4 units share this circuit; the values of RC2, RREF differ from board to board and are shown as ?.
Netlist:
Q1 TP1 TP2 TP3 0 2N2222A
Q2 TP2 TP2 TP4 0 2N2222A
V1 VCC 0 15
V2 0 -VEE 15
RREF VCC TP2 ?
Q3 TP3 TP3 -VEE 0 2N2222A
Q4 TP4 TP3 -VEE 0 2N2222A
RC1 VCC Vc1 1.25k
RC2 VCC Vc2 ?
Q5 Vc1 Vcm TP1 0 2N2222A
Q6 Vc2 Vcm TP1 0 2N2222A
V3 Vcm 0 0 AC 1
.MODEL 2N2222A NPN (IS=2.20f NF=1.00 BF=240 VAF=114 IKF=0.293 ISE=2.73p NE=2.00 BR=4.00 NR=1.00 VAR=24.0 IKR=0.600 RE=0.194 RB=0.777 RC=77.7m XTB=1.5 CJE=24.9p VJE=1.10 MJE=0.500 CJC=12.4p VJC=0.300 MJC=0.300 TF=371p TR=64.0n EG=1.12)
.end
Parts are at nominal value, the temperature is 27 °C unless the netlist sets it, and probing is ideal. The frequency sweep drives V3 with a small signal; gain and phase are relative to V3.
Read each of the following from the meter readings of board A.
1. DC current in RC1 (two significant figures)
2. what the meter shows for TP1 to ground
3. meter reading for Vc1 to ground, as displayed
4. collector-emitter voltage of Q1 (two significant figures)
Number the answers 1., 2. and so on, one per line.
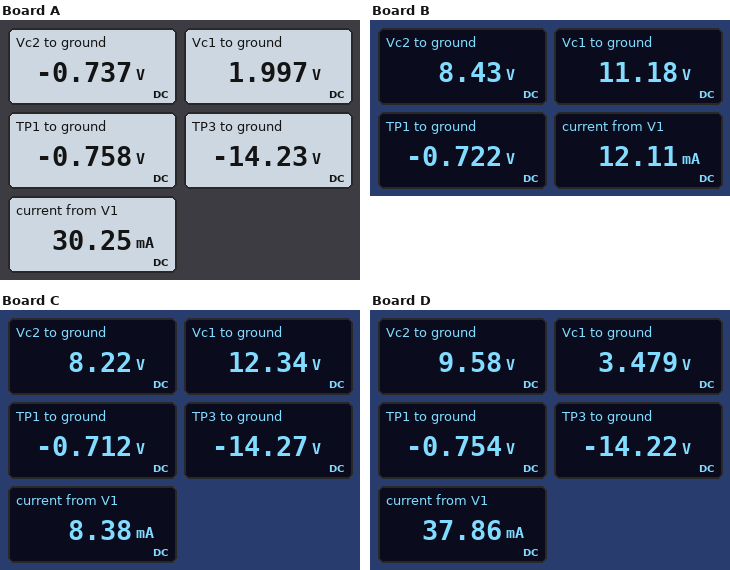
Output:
1. 10 mA
2. -0.758 V
3. 1.997 V
4. 13 V
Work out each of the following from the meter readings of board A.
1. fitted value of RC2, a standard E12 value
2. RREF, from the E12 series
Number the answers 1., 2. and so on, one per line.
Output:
1. 3.9 kΩ
2. 1.8 kΩ
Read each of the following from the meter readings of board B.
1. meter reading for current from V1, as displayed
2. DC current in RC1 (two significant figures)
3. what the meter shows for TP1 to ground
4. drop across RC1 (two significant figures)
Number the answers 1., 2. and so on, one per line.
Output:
1. 12.11 mA
2. 3.1 mA
3. -0.722 V
4. 3.8 V
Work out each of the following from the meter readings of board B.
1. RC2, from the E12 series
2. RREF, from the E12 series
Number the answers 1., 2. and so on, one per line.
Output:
1. 2.2 kΩ
2. 4.7 kΩ
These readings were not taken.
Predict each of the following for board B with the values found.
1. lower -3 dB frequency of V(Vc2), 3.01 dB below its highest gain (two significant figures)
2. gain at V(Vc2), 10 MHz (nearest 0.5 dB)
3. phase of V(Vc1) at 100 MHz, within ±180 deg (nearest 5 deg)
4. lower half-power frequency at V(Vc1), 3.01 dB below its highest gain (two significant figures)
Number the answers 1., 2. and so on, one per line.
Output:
1. 140 MHz
2. -23.0 dB
3. 85 deg
4. 140 MHz
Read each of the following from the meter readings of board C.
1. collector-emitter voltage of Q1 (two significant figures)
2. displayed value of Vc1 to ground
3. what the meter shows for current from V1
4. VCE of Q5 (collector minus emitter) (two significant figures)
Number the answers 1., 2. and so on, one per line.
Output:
1. 14 V
2. 12.34 V
3. 8.38 mA
4. 13 V
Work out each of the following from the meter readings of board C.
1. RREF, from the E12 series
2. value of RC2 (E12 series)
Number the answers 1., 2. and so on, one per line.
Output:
1. 6.8 kΩ
2. 3.3 kΩ
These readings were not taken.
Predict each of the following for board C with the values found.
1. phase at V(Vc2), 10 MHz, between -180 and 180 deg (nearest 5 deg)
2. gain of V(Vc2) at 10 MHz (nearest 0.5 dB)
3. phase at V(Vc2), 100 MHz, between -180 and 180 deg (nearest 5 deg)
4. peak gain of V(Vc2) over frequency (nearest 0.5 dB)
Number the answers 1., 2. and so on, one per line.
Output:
1. 65 deg
2. -20.0 dB
3. 60 deg
4. 0.5 dB
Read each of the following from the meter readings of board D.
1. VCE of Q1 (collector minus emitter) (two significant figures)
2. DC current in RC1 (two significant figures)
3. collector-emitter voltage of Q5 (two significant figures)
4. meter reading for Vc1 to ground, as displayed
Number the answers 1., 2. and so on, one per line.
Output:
1. 13 V
2. 9.2 mA
3. 4.2 V
4. 3.479 V
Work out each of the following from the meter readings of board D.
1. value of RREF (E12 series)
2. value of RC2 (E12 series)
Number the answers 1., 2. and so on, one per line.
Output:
1. 1.5 kΩ
2. 560 Ω
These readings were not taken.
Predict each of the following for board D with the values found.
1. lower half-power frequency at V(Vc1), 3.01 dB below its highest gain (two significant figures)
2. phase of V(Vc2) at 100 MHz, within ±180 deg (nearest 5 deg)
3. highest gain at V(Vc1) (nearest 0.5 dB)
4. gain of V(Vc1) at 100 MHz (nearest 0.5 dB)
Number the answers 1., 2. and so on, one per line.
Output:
1. 200 MHz
2. 105 deg
3. 0 dB
4. -8.0 dB
